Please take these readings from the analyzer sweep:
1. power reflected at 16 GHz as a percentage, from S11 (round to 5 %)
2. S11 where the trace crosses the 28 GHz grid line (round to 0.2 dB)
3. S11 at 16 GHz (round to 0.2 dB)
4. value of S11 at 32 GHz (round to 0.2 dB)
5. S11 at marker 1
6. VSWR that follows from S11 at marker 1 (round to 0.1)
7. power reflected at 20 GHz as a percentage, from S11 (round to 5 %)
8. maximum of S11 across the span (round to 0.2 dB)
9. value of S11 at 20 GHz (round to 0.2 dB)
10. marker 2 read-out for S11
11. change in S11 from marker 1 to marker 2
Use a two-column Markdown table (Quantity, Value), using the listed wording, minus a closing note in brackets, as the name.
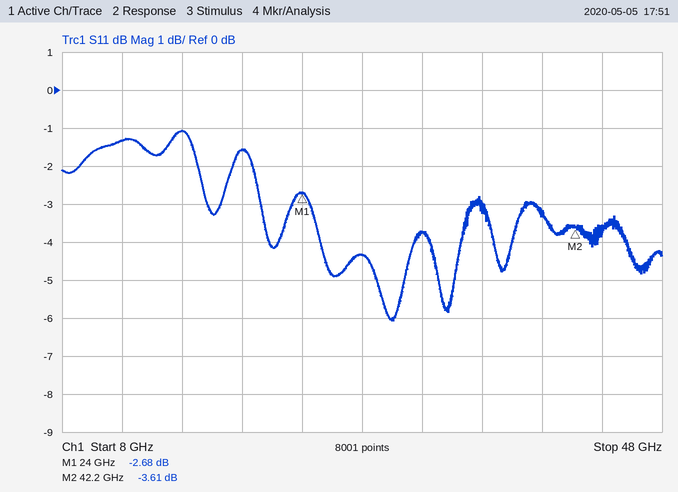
| Quantity | Value |
|---|---|
| power reflected at 16 GHz as a percentage, from S11 | 80 % |
| S11 where the trace crosses the 28 GHz grid line | -4.4 dB |
| S11 at 16 GHz | -1.0 dB |
| value of S11 at 32 GHz | -3.8 dB |
| S11 at marker 1 | -2.68 dB |
| VSWR that follows from S11 at marker 1 | 6.5 |
| power reflected at 20 GHz as a percentage, from S11 | 70 % |
| maximum of S11 across the span | -1.0 dB |
| value of S11 at 20 GHz | -1.6 dB |
| marker 2 read-out for S11 | -3.61 dB |
| change in S11 from marker 1 to marker 2 | -0.93 dB |
